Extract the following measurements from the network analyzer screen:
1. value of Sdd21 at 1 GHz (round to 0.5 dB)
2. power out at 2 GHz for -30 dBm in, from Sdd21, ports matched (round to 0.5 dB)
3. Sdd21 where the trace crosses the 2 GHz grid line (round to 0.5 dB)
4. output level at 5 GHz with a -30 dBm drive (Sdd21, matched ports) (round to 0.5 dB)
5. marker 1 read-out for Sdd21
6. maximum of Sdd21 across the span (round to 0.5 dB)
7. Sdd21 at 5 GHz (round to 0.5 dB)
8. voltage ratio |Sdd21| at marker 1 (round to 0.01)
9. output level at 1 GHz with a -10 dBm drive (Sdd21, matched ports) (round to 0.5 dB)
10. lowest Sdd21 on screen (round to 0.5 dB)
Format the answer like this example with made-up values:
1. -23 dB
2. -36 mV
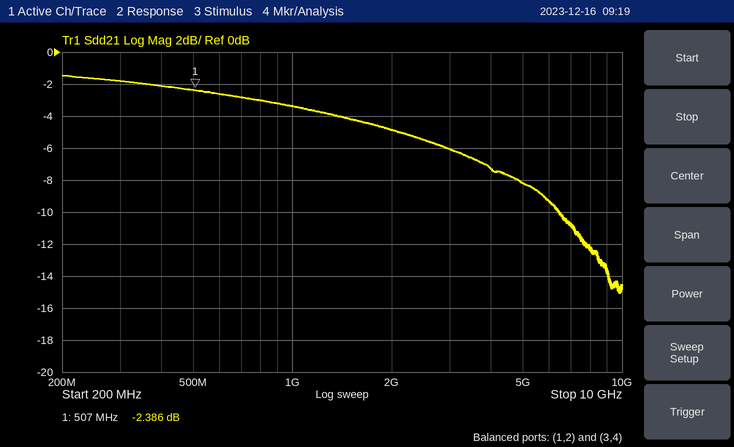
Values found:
1. -3.5 dB
2. -35.0 dBm
3. -5.0 dB
4. -38.0 dBm
5. -2.386 dB
6. -1.5 dB
7. -8.0 dB
8. 0.76
9. -13.5 dBm
10. -15.0 dB
